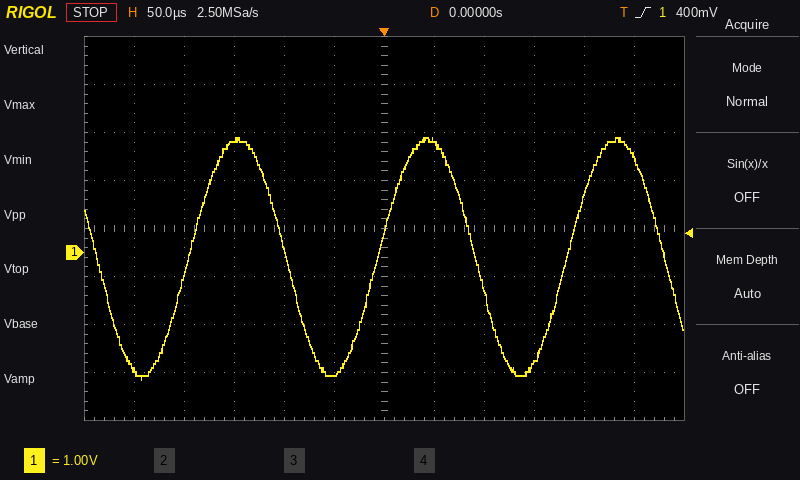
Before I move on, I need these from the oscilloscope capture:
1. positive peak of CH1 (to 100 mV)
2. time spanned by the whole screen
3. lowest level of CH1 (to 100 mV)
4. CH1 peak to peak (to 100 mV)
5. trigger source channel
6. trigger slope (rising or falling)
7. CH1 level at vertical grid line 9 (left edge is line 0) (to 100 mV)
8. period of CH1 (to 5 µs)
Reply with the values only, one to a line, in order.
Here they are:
2.4 V
600 µs
-2.6 V
5.0 V
CH1
rising
-2.3 V
190 µs
